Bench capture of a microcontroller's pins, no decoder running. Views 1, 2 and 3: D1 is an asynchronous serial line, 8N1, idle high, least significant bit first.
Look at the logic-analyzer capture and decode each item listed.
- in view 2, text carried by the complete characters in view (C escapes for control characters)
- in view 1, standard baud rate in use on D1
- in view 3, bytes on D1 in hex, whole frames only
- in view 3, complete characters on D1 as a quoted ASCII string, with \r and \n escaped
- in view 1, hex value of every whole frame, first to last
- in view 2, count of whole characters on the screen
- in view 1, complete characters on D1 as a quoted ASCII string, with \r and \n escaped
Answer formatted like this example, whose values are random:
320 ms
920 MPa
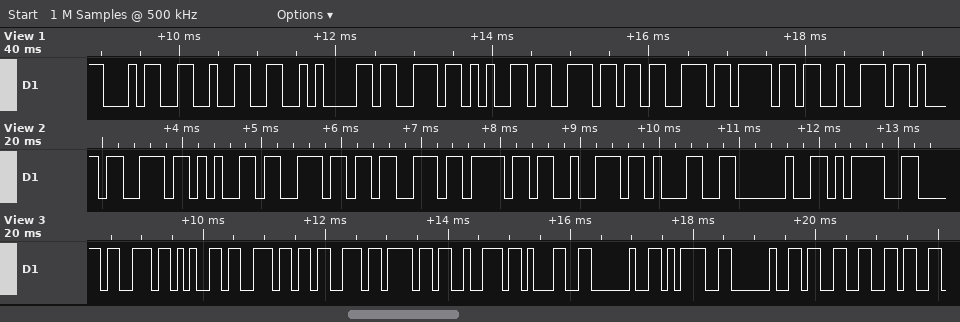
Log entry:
"sensor1 ="
9600 baud
73 65 6E 73 6F 72 31 20 3D 20 33 36
"sensor1 = 36"
34 32 0A 73 65 6E 73 6F 72
9
"42\nsensor"
